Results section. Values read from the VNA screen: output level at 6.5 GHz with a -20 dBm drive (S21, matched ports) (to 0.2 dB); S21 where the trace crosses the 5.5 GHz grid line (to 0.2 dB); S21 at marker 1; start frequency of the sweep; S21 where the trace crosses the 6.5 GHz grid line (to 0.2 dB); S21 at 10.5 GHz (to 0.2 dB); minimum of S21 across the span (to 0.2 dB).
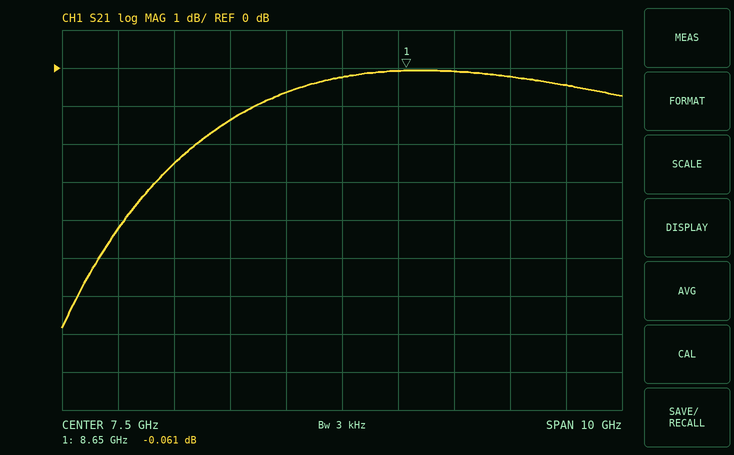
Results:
-20.6 dBm
-1.4 dB
-0.061 dB
2.5 GHz
-0.6 dB
-0.2 dB
-6.8 dB
